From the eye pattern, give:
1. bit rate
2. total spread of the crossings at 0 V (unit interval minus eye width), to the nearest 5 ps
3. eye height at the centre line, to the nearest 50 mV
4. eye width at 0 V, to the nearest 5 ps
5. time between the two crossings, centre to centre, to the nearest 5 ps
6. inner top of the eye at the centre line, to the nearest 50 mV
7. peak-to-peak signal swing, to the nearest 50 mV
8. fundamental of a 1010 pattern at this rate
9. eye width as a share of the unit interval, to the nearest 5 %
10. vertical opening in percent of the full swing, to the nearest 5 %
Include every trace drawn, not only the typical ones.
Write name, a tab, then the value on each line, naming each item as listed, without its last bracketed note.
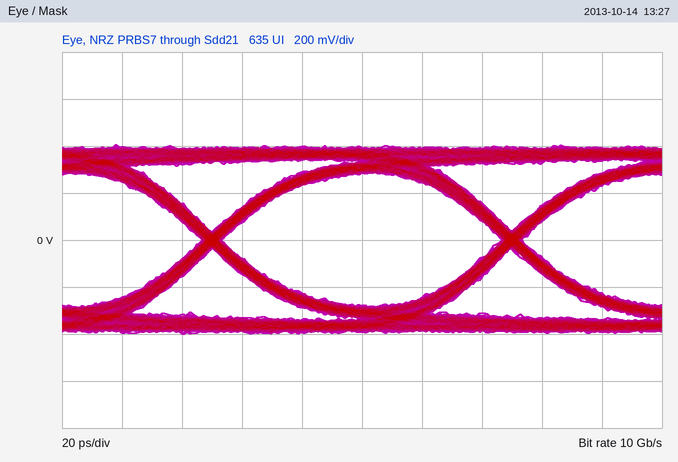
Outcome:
bit rate	10 Gb/s
total spread of the crossings at 0 V (unit interval minus eye width), to the nearest 5 ps	5 ps
eye height at the centre line, to the nearest 50 mV	550 mV
eye width at 0 V, to the nearest 5 ps	95 ps
time between the two crossings, centre to centre, to the nearest 5 ps	100 ps
inner top of the eye at the centre line, to the nearest 50 mV	300 mV
peak-to-peak signal swing, to the nearest 50 mV	800 mV
fundamental of a 1010 pattern at this rate	5 GHz
eye width as a share of the unit interval, to the nearest 5 %	95 %
vertical opening in percent of the full swing, to the nearest 5 %	70 %
